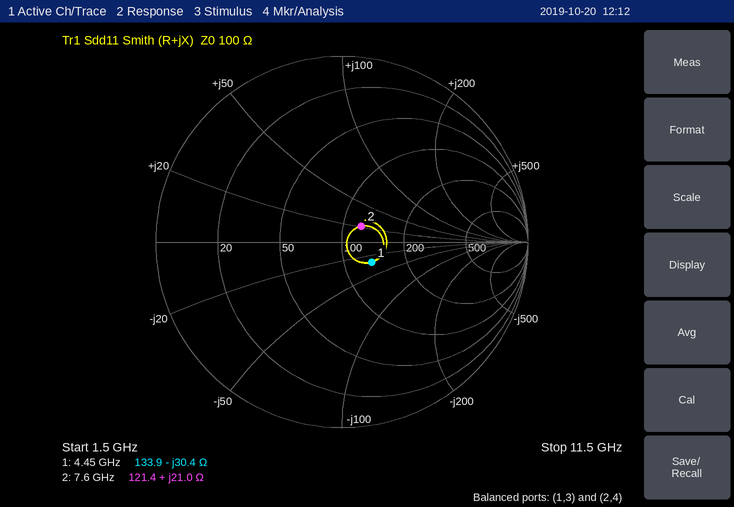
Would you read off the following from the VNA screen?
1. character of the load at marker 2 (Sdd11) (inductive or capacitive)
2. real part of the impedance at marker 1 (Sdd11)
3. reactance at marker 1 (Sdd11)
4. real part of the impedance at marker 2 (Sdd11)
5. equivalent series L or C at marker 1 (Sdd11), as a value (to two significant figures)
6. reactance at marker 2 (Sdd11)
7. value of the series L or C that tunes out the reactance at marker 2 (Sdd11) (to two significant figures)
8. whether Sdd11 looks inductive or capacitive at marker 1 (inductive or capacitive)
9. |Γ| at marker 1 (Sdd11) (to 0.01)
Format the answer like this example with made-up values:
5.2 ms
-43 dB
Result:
inductive
133.9 Ω
-30.4 Ω
121.4 Ω
1.2 pF
+21.0 Ω
1.00 pF
capacitive
0.19
